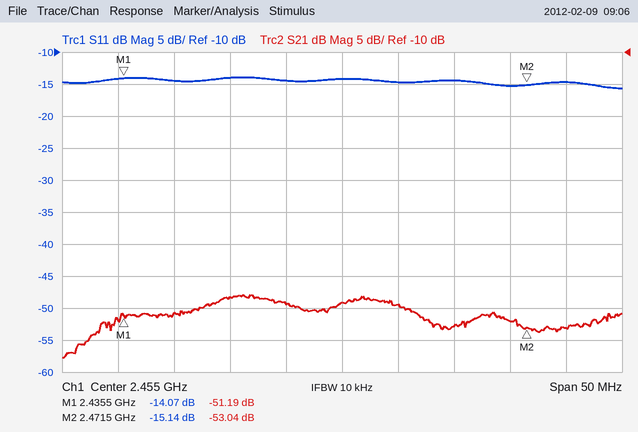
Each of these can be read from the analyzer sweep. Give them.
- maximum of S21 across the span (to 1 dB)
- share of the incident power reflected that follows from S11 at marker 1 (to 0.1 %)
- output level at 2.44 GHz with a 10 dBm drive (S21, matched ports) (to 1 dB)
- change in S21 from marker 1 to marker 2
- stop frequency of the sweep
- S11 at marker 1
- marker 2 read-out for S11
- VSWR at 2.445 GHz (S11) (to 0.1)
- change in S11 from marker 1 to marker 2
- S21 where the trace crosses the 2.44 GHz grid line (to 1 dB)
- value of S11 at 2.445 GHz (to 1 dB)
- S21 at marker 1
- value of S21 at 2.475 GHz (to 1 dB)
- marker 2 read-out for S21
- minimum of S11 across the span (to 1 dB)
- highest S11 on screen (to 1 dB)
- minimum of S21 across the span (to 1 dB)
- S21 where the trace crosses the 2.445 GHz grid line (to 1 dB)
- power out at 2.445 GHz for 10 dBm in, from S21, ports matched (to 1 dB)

-48 dB
3.9 %
-41 dBm
-1.85 dB
2.48 GHz
-14.07 dB
-15.14 dB
1.5
-1.07 dB
-51 dB
-14 dB
-51.19 dB
-53 dB
-53.04 dB
-16 dB
-14 dB
-58 dB
-48 dB
-38 dBm
